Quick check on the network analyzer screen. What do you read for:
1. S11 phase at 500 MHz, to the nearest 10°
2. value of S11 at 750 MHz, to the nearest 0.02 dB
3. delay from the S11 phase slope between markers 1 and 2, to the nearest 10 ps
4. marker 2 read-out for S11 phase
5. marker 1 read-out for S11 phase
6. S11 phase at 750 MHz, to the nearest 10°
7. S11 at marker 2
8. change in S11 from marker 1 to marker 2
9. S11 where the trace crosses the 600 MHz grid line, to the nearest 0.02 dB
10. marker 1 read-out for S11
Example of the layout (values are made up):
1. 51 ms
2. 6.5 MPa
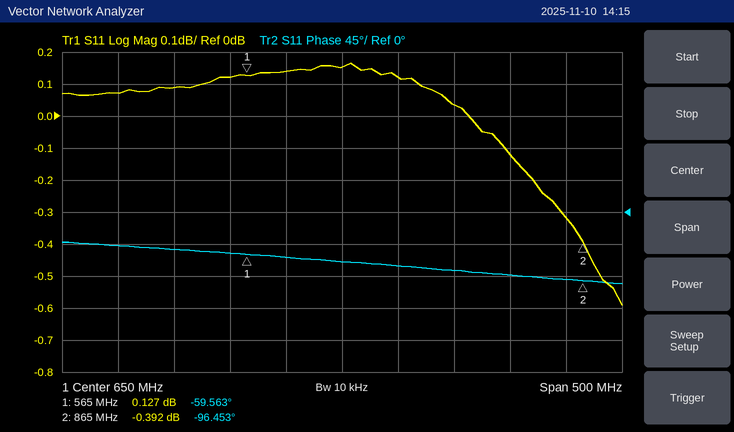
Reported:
1. -50°
2. 0.04 dB
3. 340 ps
4. -96.453°
5. -59.563°
6. -80°
7. -0.392 dB
8. -0.519 dB
9. 0.14 dB
10. 0.127 dB
